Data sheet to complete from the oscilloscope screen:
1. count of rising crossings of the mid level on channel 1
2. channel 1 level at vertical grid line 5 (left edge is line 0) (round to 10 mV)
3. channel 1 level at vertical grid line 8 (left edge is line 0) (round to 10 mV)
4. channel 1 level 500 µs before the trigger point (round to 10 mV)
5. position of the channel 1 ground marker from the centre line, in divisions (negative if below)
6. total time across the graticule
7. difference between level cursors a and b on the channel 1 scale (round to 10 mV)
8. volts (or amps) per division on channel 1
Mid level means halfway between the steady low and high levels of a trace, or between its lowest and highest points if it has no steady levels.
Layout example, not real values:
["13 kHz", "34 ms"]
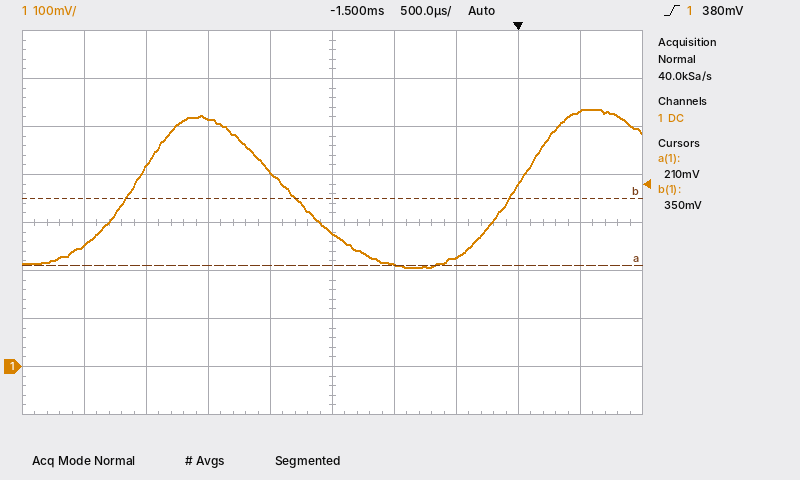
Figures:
["2", "280 mV", "380 mV", "230 mV", "-3.0 div", "5 ms", "140 mV", "100 mV"]
